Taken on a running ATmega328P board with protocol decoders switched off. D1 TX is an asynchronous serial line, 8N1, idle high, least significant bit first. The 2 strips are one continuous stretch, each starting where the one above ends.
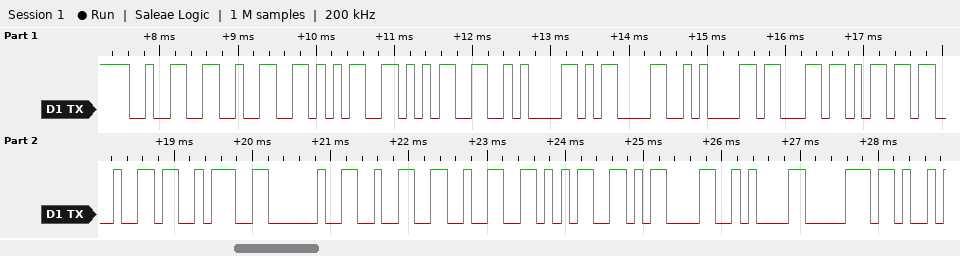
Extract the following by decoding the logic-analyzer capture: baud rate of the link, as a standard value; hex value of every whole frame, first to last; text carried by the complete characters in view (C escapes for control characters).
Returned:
9600 baud
32 32 35 35 0A 0D 0A 63 6D 64 3A 20 32 32 35 0D 0A 70
"2255\n\r\ncmd: 225\r\np"
